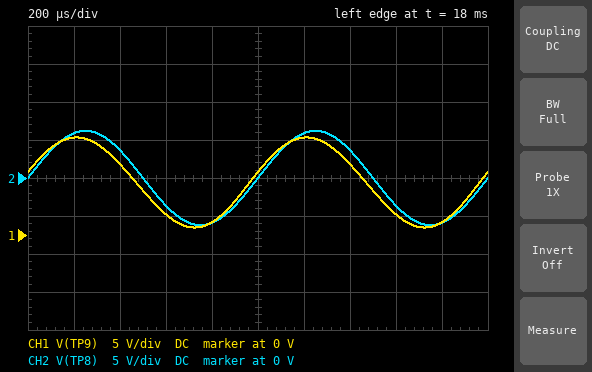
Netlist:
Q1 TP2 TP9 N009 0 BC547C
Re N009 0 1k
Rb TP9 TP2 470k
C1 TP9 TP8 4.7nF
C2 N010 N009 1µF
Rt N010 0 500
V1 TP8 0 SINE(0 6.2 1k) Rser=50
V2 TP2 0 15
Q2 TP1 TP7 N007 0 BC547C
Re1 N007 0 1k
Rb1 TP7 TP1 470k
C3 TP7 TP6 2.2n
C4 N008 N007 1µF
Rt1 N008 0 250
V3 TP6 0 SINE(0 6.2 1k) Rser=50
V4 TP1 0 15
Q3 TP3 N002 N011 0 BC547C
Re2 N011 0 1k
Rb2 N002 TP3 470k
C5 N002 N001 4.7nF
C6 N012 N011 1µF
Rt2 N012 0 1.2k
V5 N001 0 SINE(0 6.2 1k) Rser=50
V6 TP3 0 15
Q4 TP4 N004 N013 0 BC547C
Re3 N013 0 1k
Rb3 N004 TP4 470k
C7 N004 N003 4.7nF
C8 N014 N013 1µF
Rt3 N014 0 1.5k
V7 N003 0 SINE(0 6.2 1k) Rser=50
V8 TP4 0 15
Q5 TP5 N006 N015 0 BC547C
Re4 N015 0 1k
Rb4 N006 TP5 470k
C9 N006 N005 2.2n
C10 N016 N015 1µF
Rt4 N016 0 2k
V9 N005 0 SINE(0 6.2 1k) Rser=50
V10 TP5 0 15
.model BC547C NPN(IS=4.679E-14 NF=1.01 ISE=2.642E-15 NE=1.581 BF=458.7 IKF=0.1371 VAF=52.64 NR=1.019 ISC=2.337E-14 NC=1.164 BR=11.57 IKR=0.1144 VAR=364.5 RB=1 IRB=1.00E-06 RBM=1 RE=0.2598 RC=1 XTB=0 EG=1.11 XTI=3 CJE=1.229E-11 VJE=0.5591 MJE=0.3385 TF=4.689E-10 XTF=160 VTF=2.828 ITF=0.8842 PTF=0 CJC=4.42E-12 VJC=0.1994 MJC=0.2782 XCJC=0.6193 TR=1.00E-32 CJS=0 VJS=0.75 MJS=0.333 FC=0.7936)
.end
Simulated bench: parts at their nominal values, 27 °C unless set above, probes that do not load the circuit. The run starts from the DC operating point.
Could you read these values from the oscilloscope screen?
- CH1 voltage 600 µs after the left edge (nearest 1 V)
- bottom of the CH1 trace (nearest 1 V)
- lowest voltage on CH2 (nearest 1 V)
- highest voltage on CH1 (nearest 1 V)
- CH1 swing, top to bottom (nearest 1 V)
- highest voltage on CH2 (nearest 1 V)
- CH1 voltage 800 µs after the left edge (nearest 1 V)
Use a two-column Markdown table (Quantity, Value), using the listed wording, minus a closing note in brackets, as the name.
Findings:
| Quantity | Value |
|---|---|
| CH1 voltage 600 µs after the left edge | 3 V |
| bottom of the CH1 trace | 1 V |
| lowest voltage on CH2 | -6 V |
| highest voltage on CH1 | 13 V |
| CH1 swing, top to bottom | 12 V |
| highest voltage on CH2 | 6 V |
| CH1 voltage 800 µs after the left edge | 2 V |
